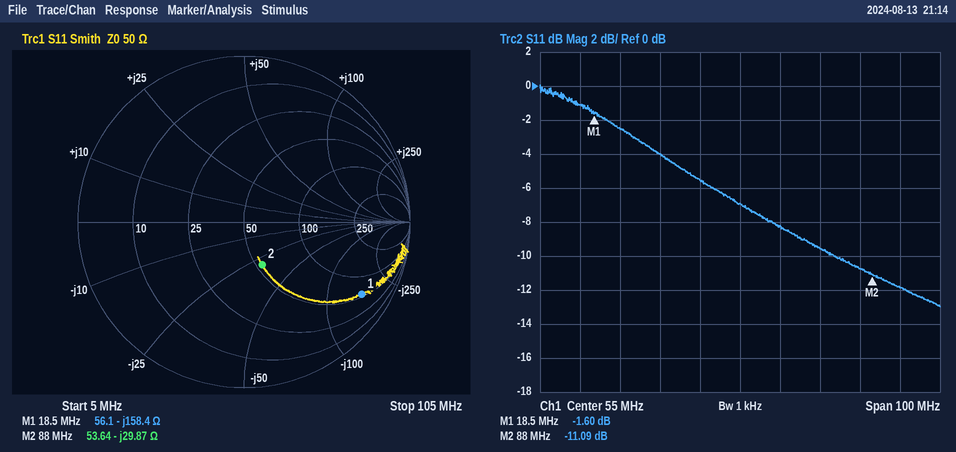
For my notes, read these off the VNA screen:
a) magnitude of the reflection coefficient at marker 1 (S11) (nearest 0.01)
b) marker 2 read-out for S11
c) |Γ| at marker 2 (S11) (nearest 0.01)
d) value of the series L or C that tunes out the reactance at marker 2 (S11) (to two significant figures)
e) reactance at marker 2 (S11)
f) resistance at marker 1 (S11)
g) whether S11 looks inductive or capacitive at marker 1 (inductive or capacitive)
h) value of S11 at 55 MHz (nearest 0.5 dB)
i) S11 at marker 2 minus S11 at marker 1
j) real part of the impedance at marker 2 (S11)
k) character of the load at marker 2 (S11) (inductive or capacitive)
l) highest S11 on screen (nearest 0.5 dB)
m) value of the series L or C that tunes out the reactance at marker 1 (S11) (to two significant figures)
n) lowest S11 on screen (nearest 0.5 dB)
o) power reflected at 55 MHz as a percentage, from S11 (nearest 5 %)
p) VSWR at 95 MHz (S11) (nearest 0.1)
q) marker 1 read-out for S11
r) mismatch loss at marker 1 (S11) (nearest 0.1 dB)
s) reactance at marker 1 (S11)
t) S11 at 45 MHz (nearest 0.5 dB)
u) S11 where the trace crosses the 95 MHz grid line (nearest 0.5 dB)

0.83
-11.09 dB
0.28
54 nH
-29.87 Ω
56.1 Ω
capacitive
-7.0 dB
-9.49 dB
53.64 Ω
capacitive
0.0 dB
1.4 µH
-13.0 dB
20 %
1.7
-1.60 dB
5.1 dB
-158.4 Ω
-5.5 dB
-12.0 dB
